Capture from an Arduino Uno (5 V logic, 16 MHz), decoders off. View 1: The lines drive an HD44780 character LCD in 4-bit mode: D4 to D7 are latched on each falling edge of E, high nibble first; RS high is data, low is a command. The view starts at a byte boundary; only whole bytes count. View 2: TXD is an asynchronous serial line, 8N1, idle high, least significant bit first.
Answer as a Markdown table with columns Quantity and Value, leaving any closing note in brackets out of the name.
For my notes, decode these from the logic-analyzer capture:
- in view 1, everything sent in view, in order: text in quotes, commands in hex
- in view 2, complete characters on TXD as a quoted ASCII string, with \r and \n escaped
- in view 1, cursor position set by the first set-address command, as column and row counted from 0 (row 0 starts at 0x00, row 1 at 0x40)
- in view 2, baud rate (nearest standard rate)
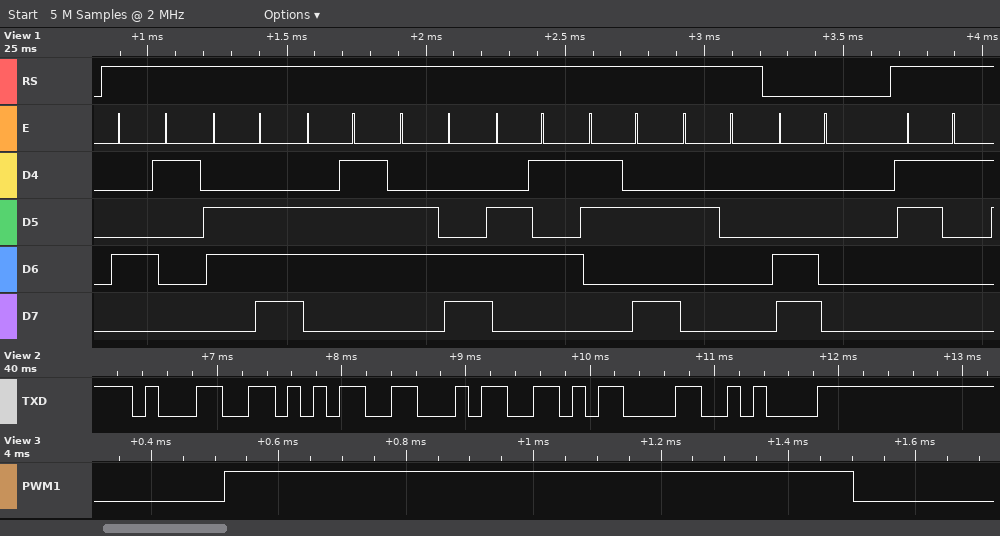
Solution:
| Quantity | Value |
|---|---|
| in view 1, everything sent in view, in order: text in quotes, commands in hex | "Angle: " 0xC0 "1" |
| in view 2, complete characters on TXD as a quoted ASCII string, with \r and \n escaped | "154\r\n" |
| in view 1, cursor position set by the first set-address command, as column and row counted from 0 | column 0, row 1 |
| in view 2, baud rate | 9600 baud |
